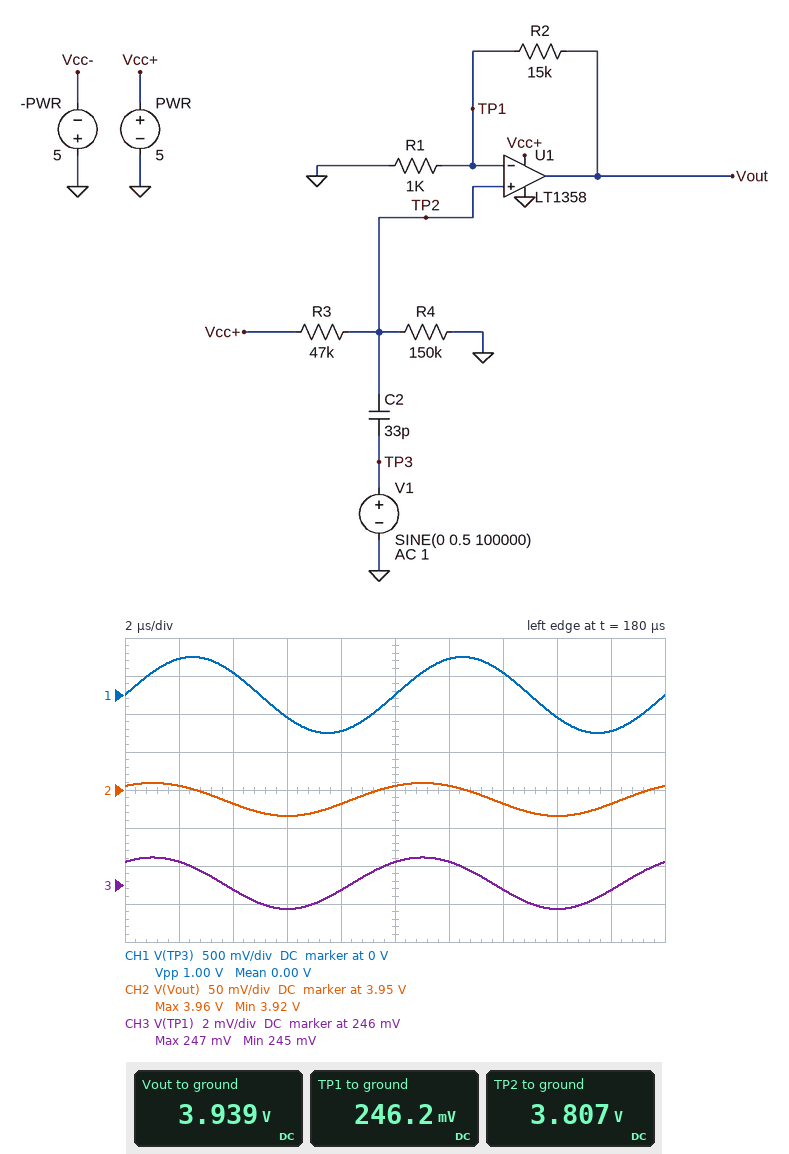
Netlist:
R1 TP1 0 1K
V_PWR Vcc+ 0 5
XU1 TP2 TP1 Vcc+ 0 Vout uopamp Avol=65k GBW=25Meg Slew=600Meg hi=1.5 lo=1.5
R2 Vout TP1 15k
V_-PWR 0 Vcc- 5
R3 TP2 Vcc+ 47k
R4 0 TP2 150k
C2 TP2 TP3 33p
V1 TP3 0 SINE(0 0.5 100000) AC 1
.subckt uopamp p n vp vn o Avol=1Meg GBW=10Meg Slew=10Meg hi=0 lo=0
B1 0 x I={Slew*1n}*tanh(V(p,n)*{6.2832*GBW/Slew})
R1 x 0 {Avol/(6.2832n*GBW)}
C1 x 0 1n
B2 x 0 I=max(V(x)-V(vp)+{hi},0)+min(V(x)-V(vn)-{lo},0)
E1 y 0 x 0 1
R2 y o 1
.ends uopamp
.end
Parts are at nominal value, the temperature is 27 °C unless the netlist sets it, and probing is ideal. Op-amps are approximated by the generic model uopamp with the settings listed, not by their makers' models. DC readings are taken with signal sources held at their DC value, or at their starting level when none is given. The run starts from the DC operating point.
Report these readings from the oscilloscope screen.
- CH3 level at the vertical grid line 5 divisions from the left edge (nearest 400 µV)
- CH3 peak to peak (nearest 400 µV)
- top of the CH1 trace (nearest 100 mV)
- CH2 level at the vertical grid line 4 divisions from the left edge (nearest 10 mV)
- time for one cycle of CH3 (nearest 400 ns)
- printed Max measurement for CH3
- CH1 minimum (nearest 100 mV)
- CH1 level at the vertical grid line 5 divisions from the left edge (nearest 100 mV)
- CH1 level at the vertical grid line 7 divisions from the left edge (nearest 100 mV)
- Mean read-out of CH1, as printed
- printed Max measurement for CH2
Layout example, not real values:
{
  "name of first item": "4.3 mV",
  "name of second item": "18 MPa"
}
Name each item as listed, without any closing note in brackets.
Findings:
{
  "CH3 level at the vertical grid line 5 divisions from the left edge": "247.2 mV",
  "CH3 peak to peak": "2.8 mV",
  "top of the CH1 trace": "500 mV",
  "CH2 level at the vertical grid line 4 divisions from the left edge": "3.93 V",
  "time for one cycle of CH3": "10.0 µs",
  "printed Max measurement for CH3": "247 mV",
  "CH1 minimum": "-500 mV",
  "CH1 level at the vertical grid line 5 divisions from the left edge": "0 V",
  "CH1 level at the vertical grid line 7 divisions from the left edge": "300 mV",
  "Mean read-out of CH1, as printed": "0.00 V",
  "printed Max measurement for CH2": "3.96 V"
}
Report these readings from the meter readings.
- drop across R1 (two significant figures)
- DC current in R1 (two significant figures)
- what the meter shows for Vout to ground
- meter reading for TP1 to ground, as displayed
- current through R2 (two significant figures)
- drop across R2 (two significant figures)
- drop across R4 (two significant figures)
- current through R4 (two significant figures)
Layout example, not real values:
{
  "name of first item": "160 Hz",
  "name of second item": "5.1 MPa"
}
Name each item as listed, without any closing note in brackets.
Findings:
{
  "drop across R1": "250 mV",
  "DC current in R1": "250 µA",
  "what the meter shows for Vout to ground": "3.939 V",
  "meter reading for TP1 to ground, as displayed": "246.2 mV",
  "current through R2": "250 µA",
  "drop across R2": "3.7 V",
  "drop across R4": "3.8 V",
  "current through R4": "25 µA"
}
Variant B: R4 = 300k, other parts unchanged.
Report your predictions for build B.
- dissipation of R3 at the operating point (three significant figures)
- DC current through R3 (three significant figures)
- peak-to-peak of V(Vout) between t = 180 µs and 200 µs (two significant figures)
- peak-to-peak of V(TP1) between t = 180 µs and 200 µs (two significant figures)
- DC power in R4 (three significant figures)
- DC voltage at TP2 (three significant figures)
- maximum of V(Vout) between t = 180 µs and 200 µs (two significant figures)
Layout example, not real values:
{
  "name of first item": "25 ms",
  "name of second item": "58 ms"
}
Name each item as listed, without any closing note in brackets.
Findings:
{
  "dissipation of R3 at the operating point": "9.76 µW",
  "DC current through R3": "14.4 µA",
  "peak-to-peak of V(Vout) between t = 180 µs and 200 µs": "38 mV",
  "peak-to-peak of V(TP1) between t = 180 µs and 200 µs": "2.4 mV",
  "DC power in R4": "62.3 µW",
  "DC voltage at TP2": "4.32 V",
  "maximum of V(Vout) between t = 180 µs and 200 µs": "4.0 V"
}
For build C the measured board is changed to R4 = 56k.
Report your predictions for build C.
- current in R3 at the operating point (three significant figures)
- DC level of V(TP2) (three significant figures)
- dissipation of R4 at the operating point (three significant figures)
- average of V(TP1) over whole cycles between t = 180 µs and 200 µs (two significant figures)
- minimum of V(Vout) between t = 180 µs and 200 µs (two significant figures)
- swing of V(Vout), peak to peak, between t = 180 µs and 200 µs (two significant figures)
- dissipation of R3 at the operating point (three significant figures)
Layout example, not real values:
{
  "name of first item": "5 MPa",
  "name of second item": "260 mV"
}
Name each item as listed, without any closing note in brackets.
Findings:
{
  "current in R3 at the operating point": "48.5 µA",
  "DC level of V(TP2)": "2.72 V",
  "dissipation of R4 at the operating point": "132 µW",
  "average of V(TP1) over whole cycles between t = 180 µs and 200 µs": "240 mV",
  "minimum of V(Vout) between t = 180 µs and 200 µs": "3.8 V",
  "swing of V(Vout), peak to peak, between t = 180 µs and 200 µs": "49 mV",
  "dissipation of R3 at the operating point": "111 µW"
}
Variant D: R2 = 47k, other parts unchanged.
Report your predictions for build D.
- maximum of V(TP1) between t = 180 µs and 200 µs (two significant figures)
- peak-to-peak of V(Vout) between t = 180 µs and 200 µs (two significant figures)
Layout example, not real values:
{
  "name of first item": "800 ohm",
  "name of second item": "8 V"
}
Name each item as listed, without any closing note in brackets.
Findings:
{
  "maximum of V(TP1) between t = 180 µs and 200 µs": "83 mV",
  "peak-to-peak of V(Vout) between t = 180 µs and 200 µs": "41 mV"
}
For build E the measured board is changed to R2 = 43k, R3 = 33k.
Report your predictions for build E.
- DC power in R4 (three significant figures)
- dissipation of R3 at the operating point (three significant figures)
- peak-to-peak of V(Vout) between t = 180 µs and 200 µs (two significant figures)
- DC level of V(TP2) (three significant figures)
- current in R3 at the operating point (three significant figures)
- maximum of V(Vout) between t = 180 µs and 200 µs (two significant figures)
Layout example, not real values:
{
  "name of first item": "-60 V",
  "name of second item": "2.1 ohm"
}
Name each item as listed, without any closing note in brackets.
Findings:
{
  "DC power in R4": "112 µW",
  "dissipation of R3 at the operating point": "24.6 µW",
  "peak-to-peak of V(Vout) between t = 180 µs and 200 µs": "30 mV",
  "DC level of V(TP2)": "4.10 V",
  "current in R3 at the operating point": "27.3 µA",
  "maximum of V(Vout) between t = 180 µs and 200 µs": "4.0 V"
}
